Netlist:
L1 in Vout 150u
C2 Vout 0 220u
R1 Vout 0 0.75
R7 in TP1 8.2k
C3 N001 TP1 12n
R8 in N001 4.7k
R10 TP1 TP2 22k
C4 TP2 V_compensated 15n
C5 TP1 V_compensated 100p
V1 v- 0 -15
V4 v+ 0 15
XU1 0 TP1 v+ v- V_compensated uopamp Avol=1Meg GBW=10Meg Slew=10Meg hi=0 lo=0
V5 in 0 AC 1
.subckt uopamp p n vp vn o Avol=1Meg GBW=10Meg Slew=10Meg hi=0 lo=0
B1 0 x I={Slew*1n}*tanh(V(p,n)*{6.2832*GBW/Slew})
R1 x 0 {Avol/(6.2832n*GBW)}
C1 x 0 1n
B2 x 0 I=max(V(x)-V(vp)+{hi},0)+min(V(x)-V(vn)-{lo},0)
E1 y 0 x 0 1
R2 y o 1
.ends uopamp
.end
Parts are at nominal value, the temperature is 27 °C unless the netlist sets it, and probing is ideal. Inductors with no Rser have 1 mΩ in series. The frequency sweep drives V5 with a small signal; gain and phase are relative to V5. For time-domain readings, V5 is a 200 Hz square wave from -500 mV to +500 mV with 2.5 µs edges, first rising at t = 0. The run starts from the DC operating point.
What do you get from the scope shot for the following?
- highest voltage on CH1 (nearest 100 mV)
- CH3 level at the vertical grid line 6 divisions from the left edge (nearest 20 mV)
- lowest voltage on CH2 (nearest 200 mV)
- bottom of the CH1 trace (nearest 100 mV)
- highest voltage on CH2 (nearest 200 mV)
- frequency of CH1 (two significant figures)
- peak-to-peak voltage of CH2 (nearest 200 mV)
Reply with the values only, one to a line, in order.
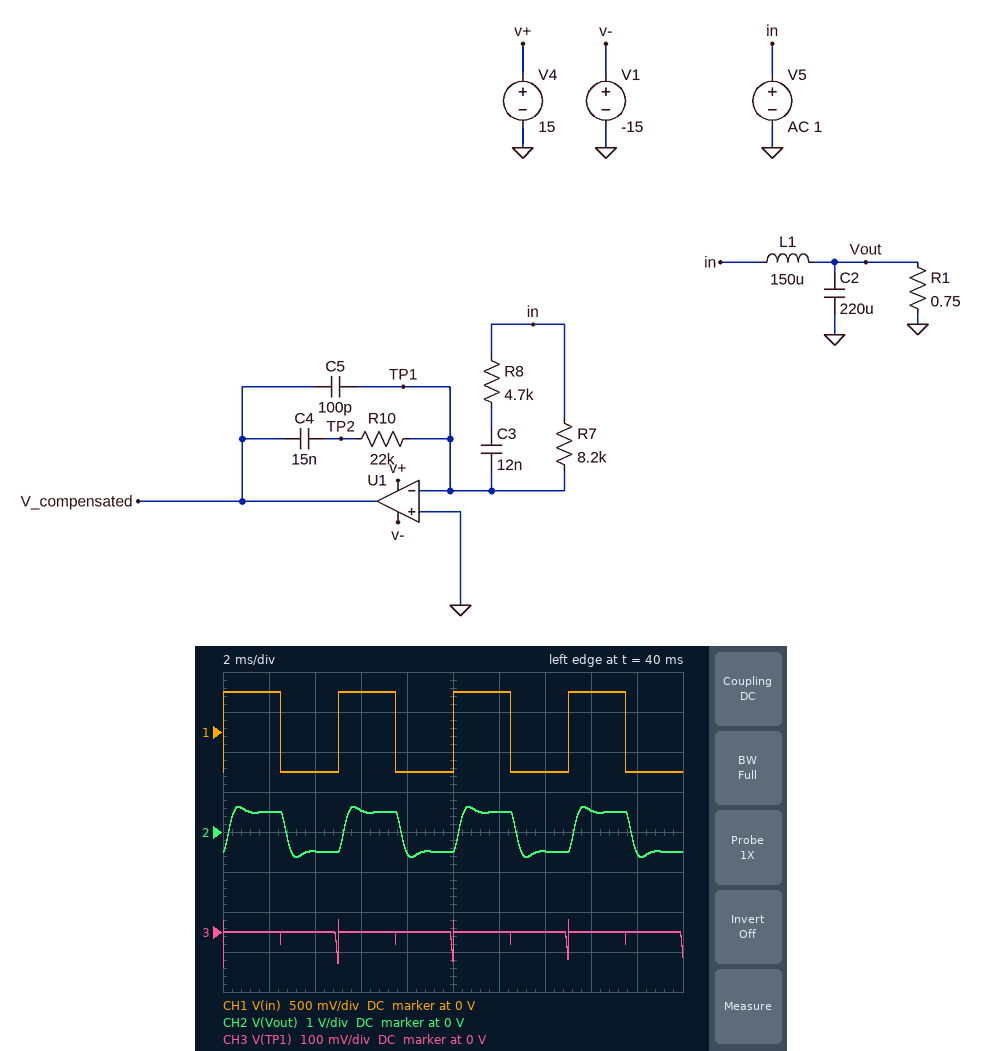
500 mV
0 V
-600 mV
-500 mV
600 mV
200 Hz
1.2 V
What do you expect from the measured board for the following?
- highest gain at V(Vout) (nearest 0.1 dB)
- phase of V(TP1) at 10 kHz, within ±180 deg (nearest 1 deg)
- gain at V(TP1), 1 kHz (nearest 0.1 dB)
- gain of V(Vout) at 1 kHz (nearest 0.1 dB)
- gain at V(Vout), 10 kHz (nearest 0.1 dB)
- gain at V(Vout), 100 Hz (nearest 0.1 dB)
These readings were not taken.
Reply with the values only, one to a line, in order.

0.7 dB
89 deg
-68.2 dB
-2.2 dB
-42.3 dB
0 dB
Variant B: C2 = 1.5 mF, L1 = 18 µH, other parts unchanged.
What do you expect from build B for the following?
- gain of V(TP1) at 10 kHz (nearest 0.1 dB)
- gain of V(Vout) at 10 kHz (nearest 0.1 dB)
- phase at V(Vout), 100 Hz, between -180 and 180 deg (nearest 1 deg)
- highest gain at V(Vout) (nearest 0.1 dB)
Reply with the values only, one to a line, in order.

-43.1 dB
-40.5 dB
-1 deg
16.2 dB
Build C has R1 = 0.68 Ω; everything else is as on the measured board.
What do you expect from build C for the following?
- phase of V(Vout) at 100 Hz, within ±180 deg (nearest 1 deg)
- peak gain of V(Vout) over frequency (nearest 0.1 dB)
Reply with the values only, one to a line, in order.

-8 deg
0.3 dB
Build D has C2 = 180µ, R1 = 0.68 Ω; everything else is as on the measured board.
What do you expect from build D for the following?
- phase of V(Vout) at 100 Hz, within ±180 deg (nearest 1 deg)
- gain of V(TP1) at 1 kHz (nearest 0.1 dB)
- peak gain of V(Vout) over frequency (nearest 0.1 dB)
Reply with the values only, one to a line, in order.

-8 deg
-68.2 dB
0 dB
